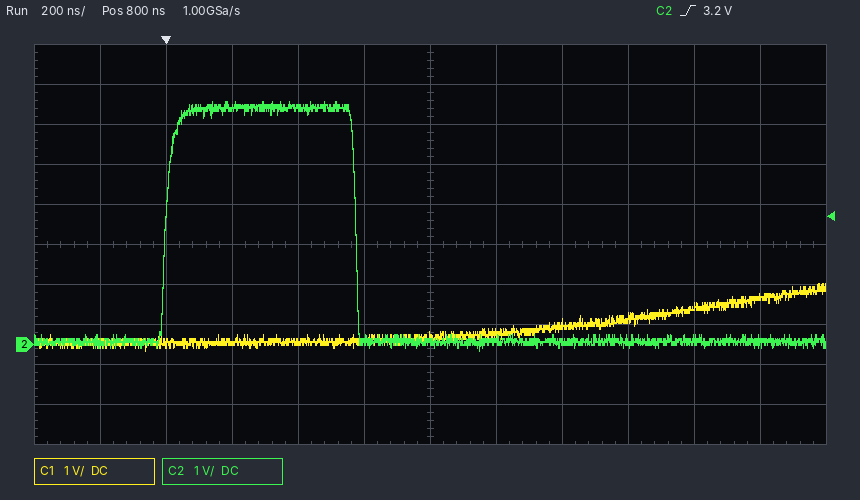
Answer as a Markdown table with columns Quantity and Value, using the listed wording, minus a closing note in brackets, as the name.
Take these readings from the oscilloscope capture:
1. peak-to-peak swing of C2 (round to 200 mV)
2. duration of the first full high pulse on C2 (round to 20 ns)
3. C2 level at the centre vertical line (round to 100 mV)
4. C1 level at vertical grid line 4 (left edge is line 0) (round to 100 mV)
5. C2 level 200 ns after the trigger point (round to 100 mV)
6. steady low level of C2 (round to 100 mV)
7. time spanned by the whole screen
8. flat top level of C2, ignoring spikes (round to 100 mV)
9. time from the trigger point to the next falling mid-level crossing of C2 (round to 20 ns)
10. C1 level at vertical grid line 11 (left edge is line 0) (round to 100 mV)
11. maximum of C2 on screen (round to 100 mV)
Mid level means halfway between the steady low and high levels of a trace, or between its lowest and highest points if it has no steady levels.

| Quantity | Value |
|---|---|
| peak-to-peak swing of C2 | 6.2 V |
| duration of the first full high pulse on C2 | 580 ns |
| C2 level at the centre vertical line | 100 mV |
| C1 level at vertical grid line 4 (left edge is line 0) | 100 mV |
| C2 level 200 ns after the trigger point | 5.9 V |
| steady low level of C2 | 100 mV |
| time spanned by the whole screen | 2.4 µs |
| flat top level of C2, ignoring spikes | 5.9 V |
| time from the trigger point to the next falling mid-level crossing of C2 | 580 ns |
| C1 level at vertical grid line 11 (left edge is line 0) | 1.2 V |
| maximum of C2 on screen | 6.1 V |
